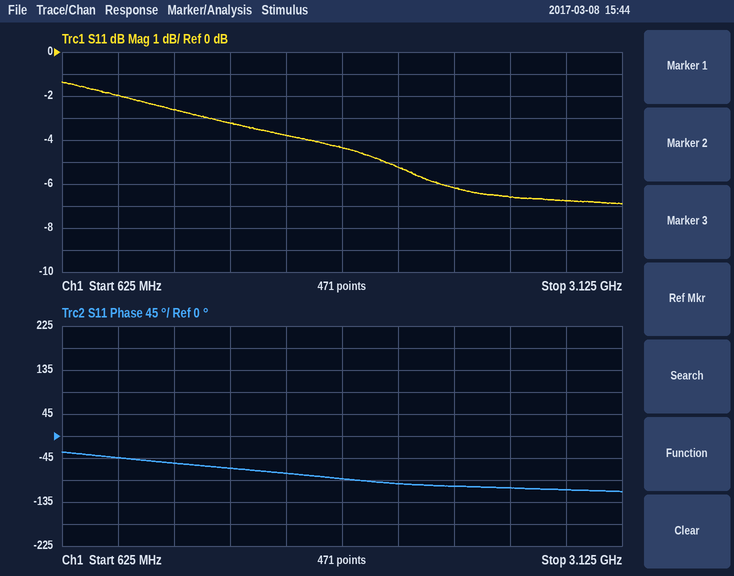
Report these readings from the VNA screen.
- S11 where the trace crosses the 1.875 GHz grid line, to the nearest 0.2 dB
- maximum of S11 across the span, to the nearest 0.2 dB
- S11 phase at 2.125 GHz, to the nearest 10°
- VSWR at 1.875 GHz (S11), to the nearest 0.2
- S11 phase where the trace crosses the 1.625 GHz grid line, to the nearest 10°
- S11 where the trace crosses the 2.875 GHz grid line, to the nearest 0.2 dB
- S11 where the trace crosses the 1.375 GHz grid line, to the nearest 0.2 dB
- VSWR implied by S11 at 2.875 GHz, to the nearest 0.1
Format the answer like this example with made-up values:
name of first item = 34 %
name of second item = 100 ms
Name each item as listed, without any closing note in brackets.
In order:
S11 where the trace crosses the 1.875 GHz grid line, to the nearest 0.2 dB = -4.4 dB
maximum of S11 across the span, to the nearest 0.2 dB = -1.4 dB
S11 phase at 2.125 GHz, to the nearest 10° = -100°
VSWR at 1.875 GHz (S11), to the nearest 0.2 = 4.0
S11 phase where the trace crosses the 1.625 GHz grid line, to the nearest 10° = -80°
S11 where the trace crosses the 2.875 GHz grid line, to the nearest 0.2 dB = -6.8 dB
S11 where the trace crosses the 1.375 GHz grid line, to the nearest 0.2 dB = -3.2 dB
VSWR implied by S11 at 2.875 GHz, to the nearest 0.1 = 2.7
